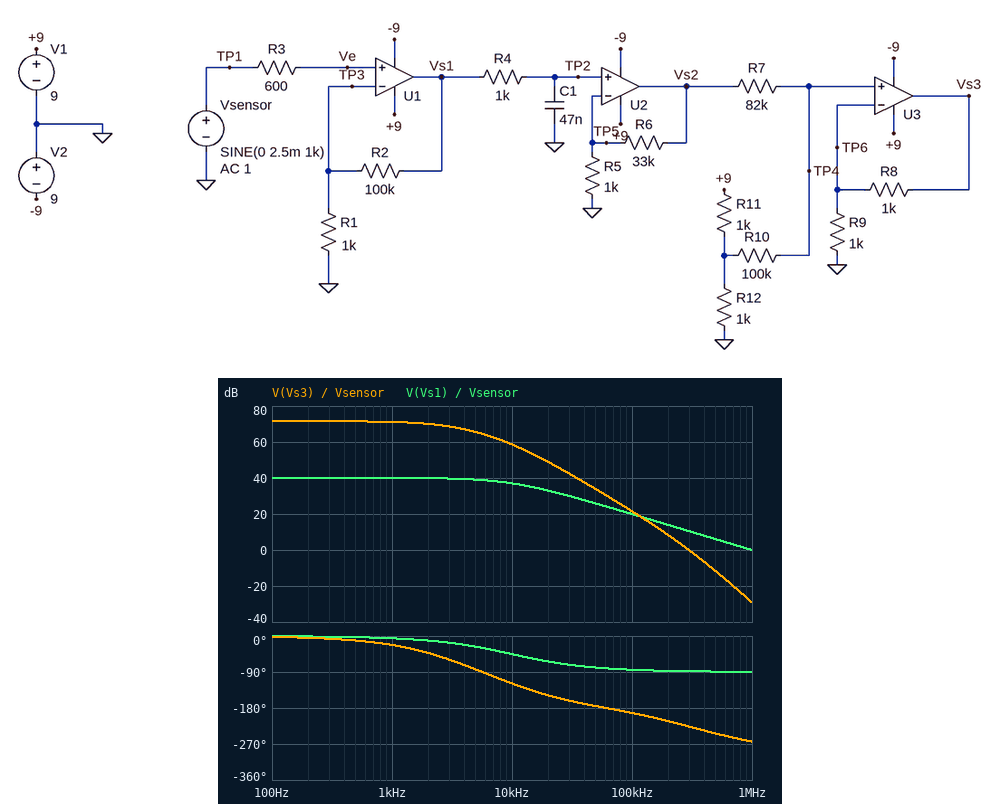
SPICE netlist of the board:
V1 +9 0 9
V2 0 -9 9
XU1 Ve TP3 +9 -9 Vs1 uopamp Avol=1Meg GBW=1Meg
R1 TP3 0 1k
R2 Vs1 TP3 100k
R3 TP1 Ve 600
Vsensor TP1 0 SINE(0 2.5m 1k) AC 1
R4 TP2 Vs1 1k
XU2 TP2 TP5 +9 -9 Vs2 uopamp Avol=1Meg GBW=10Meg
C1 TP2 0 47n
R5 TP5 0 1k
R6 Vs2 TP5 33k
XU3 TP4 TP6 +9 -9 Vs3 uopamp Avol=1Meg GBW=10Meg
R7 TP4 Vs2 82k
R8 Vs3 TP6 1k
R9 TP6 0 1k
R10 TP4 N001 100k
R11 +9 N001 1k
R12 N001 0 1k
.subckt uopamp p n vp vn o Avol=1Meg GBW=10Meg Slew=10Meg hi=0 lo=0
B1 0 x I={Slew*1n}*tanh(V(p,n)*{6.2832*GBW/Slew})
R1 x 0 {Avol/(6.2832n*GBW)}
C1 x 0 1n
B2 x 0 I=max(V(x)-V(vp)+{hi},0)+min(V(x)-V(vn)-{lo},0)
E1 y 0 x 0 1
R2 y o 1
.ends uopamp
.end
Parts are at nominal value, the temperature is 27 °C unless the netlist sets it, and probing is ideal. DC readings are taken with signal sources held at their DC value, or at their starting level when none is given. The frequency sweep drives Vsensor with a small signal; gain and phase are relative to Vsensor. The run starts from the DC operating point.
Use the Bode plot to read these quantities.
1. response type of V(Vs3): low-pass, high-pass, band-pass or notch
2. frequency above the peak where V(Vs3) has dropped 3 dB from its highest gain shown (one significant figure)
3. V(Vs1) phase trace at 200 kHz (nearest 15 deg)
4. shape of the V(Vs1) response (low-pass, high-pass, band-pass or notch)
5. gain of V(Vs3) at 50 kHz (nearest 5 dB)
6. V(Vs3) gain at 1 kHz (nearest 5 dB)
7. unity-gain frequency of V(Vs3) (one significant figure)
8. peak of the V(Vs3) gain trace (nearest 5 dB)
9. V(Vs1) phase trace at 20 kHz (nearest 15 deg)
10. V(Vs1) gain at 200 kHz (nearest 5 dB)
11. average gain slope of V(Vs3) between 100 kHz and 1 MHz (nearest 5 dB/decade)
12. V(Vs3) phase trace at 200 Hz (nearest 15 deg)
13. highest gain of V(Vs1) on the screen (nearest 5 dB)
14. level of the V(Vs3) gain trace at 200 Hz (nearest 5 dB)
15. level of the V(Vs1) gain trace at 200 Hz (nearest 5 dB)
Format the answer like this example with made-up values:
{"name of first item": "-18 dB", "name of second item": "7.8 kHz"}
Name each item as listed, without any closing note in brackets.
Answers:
{"response type of V(Vs3): low-pass, high-pass, band-pass or notch": "low-pass", "frequency above the peak where V(Vs3) has dropped 3 dB from its highest gain shown": "3 kHz", "V(Vs1) phase trace at 200 kHz": "-90 deg", "shape of the V(Vs1) response": "low-pass", "gain of V(Vs3) at 50 kHz": "35 dB", "V(Vs3) gain at 1 kHz": "70 dB", "unity-gain frequency of V(Vs3)": "300 kHz", "peak of the V(Vs3) gain trace": "70 dB", "V(Vs1) phase trace at 20 kHz": "-60 deg", "V(Vs1) gain at 200 kHz": "15 dB", "average gain slope of V(Vs3) between 100 kHz and 1 MHz": "-50 dB/decade", "V(Vs3) phase trace at 200 Hz": "0 deg", "highest gain of V(Vs1) on the screen": "40 dB", "level of the V(Vs3) gain trace at 200 Hz": "70 dB", "level of the V(Vs1) gain trace at 200 Hz": "40 dB"}
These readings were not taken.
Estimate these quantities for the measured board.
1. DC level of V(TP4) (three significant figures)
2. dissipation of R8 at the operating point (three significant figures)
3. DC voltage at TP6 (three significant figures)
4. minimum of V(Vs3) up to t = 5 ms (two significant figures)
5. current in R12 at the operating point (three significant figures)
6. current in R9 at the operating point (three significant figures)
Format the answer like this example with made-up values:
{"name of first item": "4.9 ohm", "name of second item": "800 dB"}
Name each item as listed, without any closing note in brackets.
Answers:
{"DC level of V(TP4)": "2.02 V", "dissipation of R8 at the operating point": "4.09 mW", "DC voltage at TP6": "2.02 V", "minimum of V(Vs3) up to t = 5 ms": "-5.0 V", "current in R12 at the operating point": "4.49 mA", "current in R9 at the operating point": "2.02 mA"}
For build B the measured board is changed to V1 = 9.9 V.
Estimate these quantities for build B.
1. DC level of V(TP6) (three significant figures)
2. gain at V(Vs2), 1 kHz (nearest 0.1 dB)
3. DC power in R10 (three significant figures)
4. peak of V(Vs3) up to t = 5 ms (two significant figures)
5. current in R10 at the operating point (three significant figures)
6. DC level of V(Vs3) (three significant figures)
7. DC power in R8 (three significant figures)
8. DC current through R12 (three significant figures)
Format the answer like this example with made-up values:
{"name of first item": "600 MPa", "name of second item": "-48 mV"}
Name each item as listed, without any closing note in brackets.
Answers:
{"DC level of V(TP6)": "2.22 V", "gain at V(Vs2), 1 kHz": "70.3 dB", "DC power in R10": "73.6 µW", "peak of V(Vs3) up to t = 5 ms": "9.9 V", "current in R10 at the operating point": "27.1 µA", "DC level of V(Vs3)": "4.45 V", "DC power in R8": "4.95 mW", "DC current through R12": "4.94 mA"}
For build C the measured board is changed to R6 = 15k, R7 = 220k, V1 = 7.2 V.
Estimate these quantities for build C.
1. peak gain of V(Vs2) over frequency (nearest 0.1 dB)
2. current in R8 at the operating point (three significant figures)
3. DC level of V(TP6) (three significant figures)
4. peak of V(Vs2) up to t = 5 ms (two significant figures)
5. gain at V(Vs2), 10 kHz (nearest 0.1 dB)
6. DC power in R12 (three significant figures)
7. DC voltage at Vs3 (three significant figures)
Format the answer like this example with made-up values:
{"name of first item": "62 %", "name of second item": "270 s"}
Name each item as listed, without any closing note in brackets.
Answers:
{"peak gain of V(Vs2) over frequency": "64.2 dB", "current in R8 at the operating point": "2.47 mA", "DC level of V(TP6)": "2.47 V", "peak of V(Vs2) up to t = 5 ms": "3.9 V", "gain at V(Vs2), 10 kHz": "51.2 dB", "DC power in R12": "12.9 mW", "DC voltage at Vs3": "4.94 V"}
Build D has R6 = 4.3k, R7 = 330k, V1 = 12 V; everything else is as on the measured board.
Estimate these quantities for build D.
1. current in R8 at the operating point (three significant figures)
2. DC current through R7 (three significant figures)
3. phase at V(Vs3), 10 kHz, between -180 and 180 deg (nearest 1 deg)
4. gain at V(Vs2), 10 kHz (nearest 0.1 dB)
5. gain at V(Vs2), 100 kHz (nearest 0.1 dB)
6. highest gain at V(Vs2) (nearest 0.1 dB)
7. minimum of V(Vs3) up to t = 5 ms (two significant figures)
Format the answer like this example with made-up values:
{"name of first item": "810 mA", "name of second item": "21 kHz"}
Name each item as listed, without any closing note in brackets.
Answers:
{"current in R8 at the operating point": "4.60 mA", "DC current through R7": "13.9 µA", "phase at V(Vs3), 10 kHz, between -180 and 180 deg": "-117 deg", "gain at V(Vs2), 10 kHz": "41.6 dB", "gain at V(Vs2), 100 kHz": "5.0 dB", "highest gain at V(Vs2)": "54.6 dB", "minimum of V(Vs3) up to t = 5 ms": "8.6 V"}
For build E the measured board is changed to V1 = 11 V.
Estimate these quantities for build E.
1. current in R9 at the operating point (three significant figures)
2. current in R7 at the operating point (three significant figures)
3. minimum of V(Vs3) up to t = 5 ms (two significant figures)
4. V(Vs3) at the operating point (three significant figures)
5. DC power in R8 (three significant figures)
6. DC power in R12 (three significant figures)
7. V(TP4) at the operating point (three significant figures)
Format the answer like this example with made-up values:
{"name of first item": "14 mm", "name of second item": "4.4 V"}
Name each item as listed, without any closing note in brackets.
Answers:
{"current in R9 at the operating point": "2.47 mA", "current in R7 at the operating point": "30.1 µA", "minimum of V(Vs3) up to t = 5 ms": "-4.1 V", "V(Vs3) at the operating point": "4.94 V", "DC power in R8": "6.11 mW", "DC power in R12": "30.1 mW", "V(TP4) at the operating point": "2.47 V"}
